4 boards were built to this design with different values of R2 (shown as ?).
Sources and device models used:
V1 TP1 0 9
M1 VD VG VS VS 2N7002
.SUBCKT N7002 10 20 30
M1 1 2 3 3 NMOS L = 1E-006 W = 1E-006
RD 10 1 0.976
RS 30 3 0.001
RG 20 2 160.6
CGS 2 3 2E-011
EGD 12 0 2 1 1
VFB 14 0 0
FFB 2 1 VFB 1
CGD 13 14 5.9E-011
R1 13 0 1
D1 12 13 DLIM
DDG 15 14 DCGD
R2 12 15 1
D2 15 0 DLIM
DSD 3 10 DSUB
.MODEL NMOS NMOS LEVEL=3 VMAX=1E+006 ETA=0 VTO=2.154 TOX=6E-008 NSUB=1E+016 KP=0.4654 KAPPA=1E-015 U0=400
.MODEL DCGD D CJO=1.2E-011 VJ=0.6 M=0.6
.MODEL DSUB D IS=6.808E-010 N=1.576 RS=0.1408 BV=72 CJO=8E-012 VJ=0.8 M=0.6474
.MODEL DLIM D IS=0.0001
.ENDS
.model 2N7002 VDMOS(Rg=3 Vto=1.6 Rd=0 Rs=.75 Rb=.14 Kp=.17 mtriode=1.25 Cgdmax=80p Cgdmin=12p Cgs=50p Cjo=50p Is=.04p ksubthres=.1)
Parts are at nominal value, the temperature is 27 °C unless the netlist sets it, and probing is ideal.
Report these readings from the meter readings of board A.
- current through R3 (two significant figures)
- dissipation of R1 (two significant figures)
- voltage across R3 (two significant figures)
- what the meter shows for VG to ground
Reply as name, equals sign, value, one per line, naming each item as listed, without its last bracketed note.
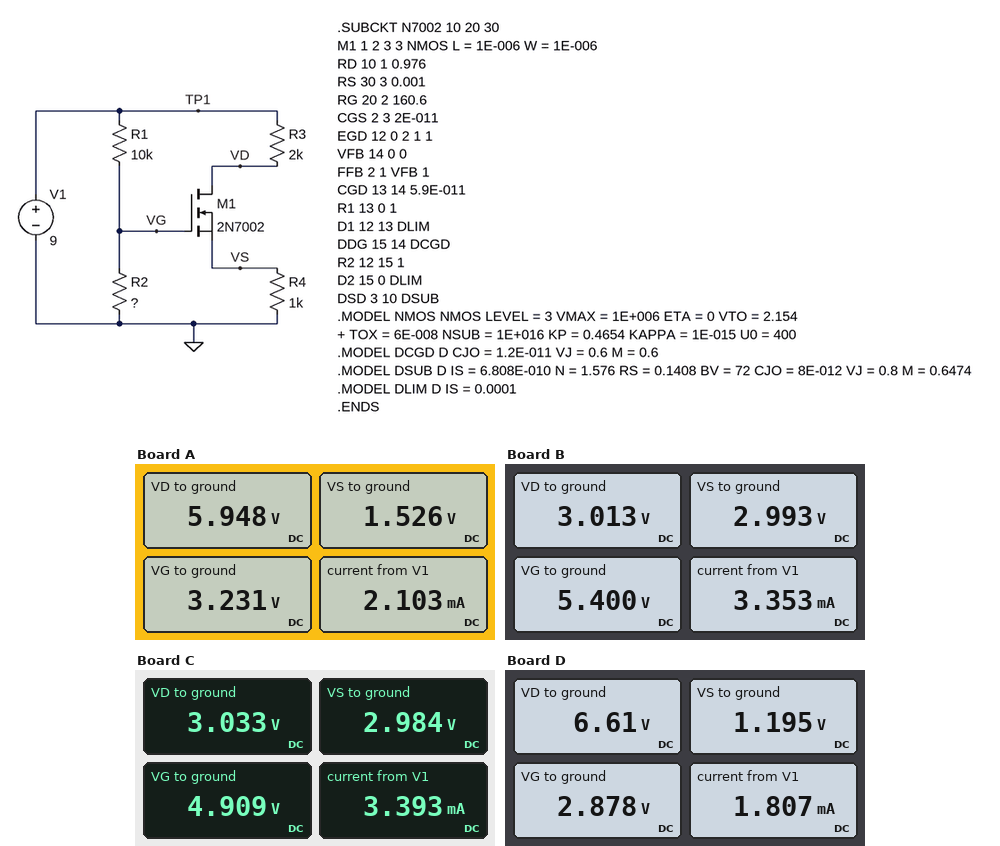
current through R3 = 1.5 mA
dissipation of R1 = 3.3 mW
voltage across R3 = 3.1 V
what the meter shows for VG to ground = 3.231 V
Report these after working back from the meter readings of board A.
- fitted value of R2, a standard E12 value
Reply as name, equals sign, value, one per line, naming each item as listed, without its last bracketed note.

fitted value of R2, a standard E12 value = 5.6 kΩ
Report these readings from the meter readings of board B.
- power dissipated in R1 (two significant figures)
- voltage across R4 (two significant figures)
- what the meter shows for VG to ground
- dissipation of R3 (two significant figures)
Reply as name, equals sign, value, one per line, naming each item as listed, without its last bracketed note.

power dissipated in R1 = 1.3 mW
voltage across R4 = 3.0 V
what the meter shows for VG to ground = 5.400 V
dissipation of R3 = 18 mW
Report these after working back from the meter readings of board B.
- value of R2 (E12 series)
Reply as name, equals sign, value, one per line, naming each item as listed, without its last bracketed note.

value of R2 = 15 kΩ
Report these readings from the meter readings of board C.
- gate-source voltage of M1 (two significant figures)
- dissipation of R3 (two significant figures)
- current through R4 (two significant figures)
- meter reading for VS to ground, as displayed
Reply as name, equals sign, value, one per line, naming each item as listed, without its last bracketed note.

gate-source voltage of M1 = 1.9 V
dissipation of R3 = 18 mW
current through R4 = 3.0 mA
meter reading for VS to ground, as displayed = 2.984 V
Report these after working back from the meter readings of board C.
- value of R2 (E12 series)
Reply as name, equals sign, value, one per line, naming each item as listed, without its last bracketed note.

value of R2 = 12 kΩ
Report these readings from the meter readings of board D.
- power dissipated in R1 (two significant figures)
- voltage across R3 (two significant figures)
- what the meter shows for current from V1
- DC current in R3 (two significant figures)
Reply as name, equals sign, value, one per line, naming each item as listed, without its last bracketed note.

power dissipated in R1 = 3.7 mW
voltage across R3 = 2.4 V
what the meter shows for current from V1 = 1.807 mA
DC current in R3 = 1.2 mA
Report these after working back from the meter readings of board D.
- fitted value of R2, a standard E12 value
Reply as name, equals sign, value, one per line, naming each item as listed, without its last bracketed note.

fitted value of R2, a standard E12 value = 4.7 kΩ
